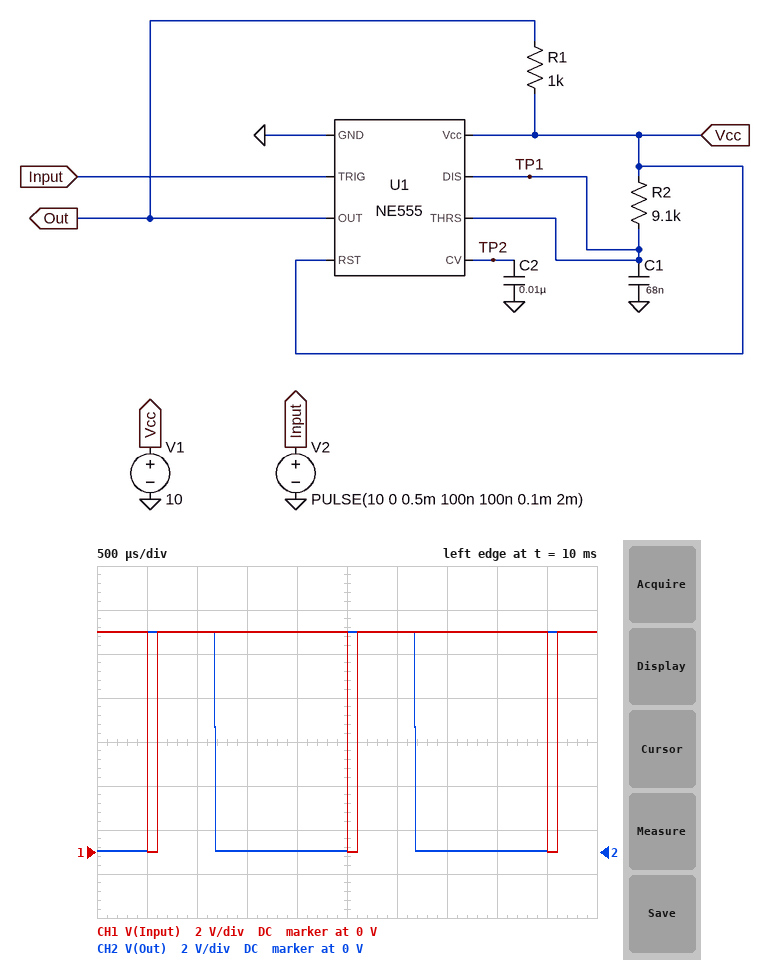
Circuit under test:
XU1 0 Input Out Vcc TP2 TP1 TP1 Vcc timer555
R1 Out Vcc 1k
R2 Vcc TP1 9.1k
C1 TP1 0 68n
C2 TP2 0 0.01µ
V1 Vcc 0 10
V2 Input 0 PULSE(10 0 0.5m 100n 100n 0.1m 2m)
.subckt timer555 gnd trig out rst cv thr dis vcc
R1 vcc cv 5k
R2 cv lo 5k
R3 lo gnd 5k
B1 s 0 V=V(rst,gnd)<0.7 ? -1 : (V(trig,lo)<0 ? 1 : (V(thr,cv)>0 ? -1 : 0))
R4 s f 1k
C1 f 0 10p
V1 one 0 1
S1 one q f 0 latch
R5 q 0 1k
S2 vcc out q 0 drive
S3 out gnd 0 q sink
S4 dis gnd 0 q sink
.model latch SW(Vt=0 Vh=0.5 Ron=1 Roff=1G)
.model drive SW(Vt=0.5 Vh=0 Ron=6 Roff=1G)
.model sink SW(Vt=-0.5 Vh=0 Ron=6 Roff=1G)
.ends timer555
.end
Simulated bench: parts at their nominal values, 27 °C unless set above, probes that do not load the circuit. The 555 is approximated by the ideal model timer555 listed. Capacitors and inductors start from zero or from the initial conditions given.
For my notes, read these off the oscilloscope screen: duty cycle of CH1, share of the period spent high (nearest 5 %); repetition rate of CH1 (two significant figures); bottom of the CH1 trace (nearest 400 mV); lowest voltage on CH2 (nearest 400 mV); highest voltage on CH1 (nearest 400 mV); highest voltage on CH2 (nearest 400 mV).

95 %
500 Hz
0 V
0 V
10.0 V
10.0 V
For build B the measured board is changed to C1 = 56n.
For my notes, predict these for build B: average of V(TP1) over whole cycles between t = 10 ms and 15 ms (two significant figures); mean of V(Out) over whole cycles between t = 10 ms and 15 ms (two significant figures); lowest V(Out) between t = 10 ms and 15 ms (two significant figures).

1.1 V
2.8 V
60 mV
